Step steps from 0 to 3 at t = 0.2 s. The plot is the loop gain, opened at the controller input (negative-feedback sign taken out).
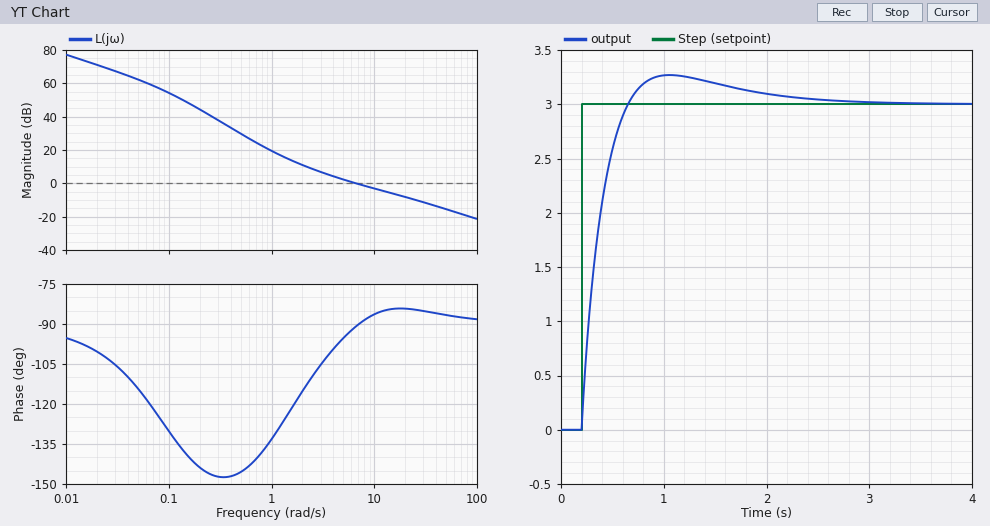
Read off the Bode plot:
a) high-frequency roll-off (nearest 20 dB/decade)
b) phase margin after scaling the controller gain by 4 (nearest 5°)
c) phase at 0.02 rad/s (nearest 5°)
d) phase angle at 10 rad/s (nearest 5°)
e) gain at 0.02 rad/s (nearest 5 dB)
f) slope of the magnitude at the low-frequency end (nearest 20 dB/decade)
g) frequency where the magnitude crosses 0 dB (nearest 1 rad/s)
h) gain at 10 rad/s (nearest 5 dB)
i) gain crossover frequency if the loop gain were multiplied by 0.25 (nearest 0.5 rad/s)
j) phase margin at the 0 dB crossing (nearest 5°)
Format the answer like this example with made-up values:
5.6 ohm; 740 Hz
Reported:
-20 dB/decade; 95°; -100°; -85°; 70 dB; -20 dB/decade; 7 rad/s; -5 dB; 2.0 rad/s; 90°
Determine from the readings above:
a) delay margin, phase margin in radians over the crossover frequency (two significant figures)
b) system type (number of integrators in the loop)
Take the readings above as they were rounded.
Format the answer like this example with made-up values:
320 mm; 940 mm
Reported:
0.22 s; 1
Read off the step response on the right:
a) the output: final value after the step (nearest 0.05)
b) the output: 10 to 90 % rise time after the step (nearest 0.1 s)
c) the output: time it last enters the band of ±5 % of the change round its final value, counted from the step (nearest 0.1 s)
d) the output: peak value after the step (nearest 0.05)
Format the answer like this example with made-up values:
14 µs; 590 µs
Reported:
3.00; 0.3 s; 1.5 s; 3.25
